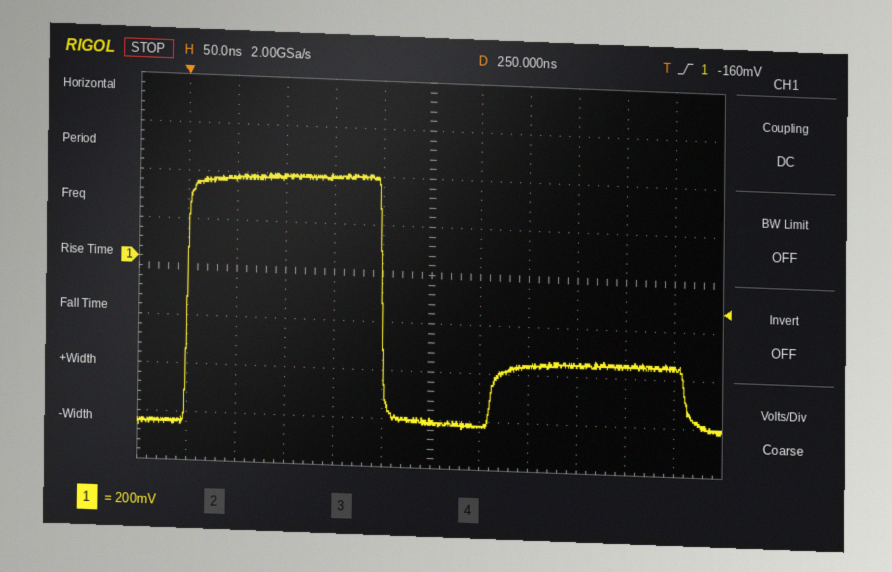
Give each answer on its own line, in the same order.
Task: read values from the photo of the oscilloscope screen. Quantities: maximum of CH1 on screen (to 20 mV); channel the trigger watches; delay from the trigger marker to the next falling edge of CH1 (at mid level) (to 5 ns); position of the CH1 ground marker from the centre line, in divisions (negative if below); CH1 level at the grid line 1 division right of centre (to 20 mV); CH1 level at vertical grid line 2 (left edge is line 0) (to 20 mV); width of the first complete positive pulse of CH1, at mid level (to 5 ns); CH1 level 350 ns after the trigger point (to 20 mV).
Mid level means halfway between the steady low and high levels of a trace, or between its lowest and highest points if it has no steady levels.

360 mV
CH1
200 ns
+0.2 div
-660 mV
340 mV
200 ns
-400 mV
